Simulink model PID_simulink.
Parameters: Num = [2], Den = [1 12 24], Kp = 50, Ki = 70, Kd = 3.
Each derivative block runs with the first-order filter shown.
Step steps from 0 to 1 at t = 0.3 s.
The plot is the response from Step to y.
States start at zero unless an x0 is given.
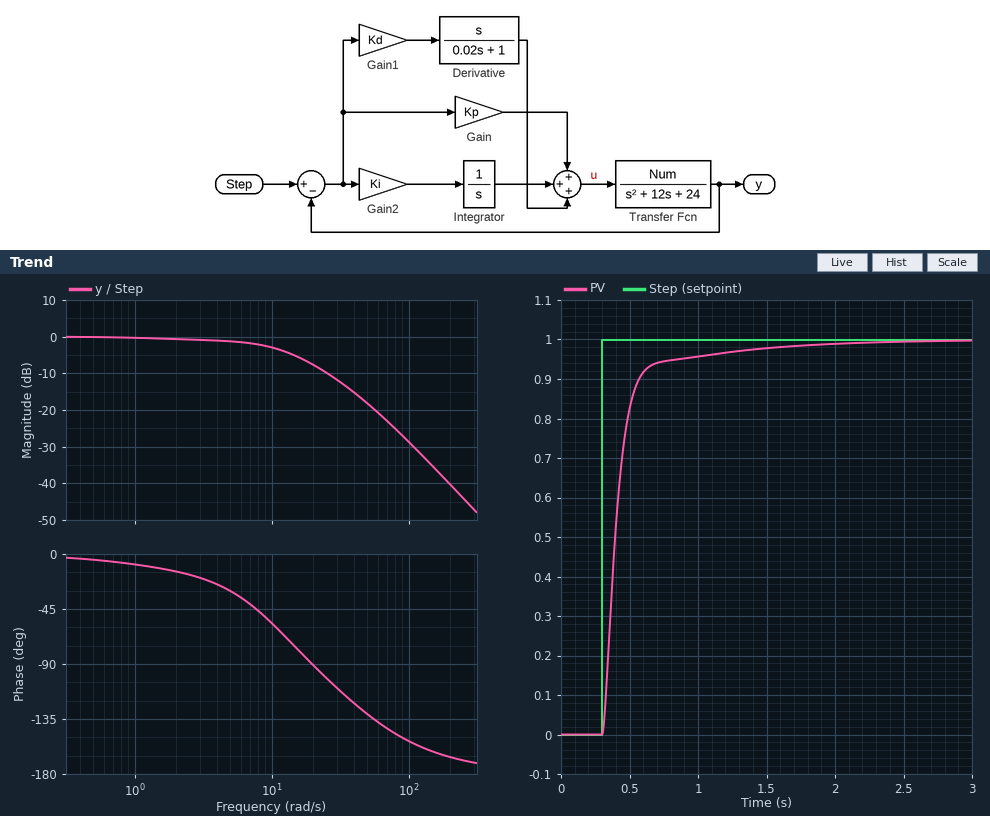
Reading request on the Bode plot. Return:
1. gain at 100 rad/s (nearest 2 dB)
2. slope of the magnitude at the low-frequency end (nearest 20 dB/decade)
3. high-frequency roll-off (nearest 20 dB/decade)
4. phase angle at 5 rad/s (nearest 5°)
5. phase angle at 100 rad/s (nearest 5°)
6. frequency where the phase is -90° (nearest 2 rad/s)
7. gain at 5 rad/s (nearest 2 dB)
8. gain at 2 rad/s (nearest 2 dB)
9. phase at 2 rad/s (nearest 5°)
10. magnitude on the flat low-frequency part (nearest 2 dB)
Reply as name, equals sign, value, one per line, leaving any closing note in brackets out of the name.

gain at 100 rad/s = -28 dB
slope of the magnitude at the low-frequency end = 0 dB/decade
high-frequency roll-off = -40 dB/decade
phase angle at 5 rad/s = -30°
phase angle at 100 rad/s = -155°
frequency where the phase is -90° = 20 rad/s
gain at 5 rad/s = -2 dB
gain at 2 rad/s = 0 dB
phase at 2 rad/s = -15°
magnitude on the flat low-frequency part = 0 dB
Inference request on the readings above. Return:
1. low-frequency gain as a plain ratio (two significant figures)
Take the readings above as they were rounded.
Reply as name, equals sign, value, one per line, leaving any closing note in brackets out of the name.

low-frequency gain as a plain ratio = 1.0
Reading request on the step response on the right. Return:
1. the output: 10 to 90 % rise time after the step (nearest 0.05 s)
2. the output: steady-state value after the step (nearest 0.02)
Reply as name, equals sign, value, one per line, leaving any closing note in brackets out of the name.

the output: 10 to 90 % rise time after the step = 0.25 s
the output: steady-state value after the step = 1.00
